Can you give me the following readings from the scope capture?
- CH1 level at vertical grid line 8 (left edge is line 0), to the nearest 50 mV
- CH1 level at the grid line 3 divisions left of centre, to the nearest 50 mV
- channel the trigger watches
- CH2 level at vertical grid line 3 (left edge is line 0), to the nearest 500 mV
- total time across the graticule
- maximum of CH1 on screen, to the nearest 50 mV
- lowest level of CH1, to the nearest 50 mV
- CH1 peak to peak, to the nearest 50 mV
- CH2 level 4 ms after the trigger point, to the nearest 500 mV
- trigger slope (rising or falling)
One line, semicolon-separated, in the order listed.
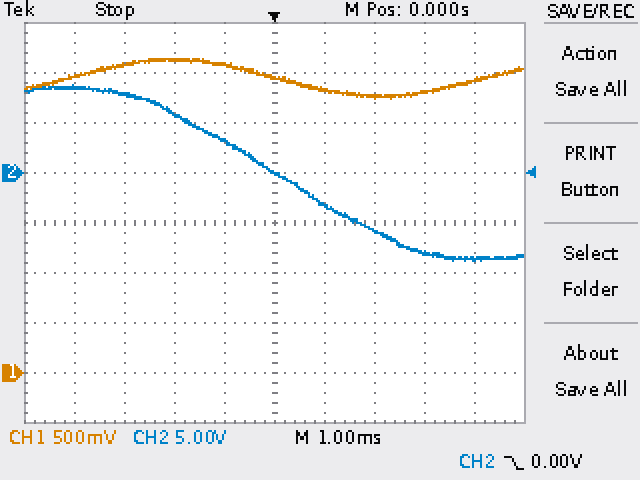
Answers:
2.80 V; 3.10 V; CH2; 6.0 V; 10 ms; 3.15 V; 2.75 V; 400 mV; -8.5 V; falling
